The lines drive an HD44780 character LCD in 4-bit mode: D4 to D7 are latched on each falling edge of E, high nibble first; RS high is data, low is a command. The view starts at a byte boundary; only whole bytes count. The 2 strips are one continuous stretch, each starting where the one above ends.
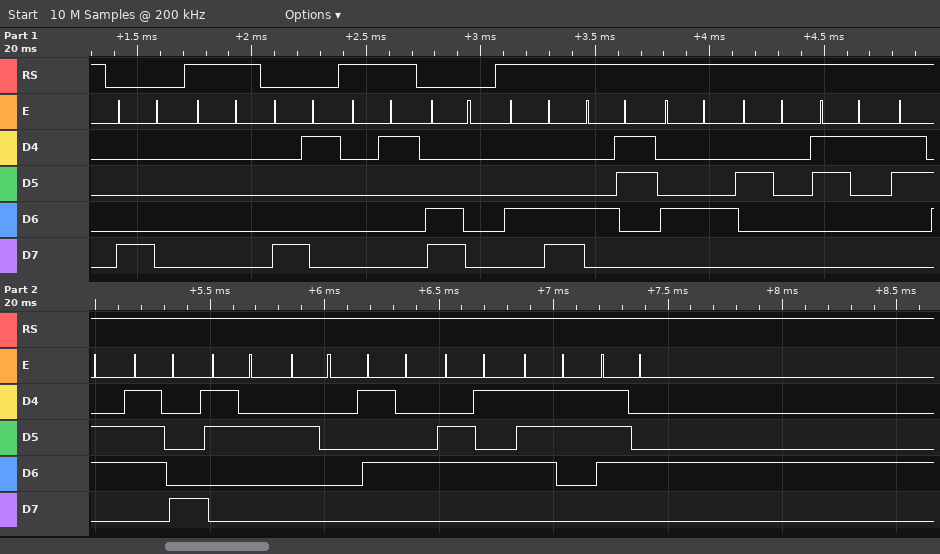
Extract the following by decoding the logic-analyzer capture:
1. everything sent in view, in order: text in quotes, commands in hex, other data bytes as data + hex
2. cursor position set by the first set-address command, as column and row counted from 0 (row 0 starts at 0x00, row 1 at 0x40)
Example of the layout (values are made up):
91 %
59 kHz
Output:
0x80 data 00 0x81 data 01 0xC0 "LCD 16x2 Test"
column 0, row 0
